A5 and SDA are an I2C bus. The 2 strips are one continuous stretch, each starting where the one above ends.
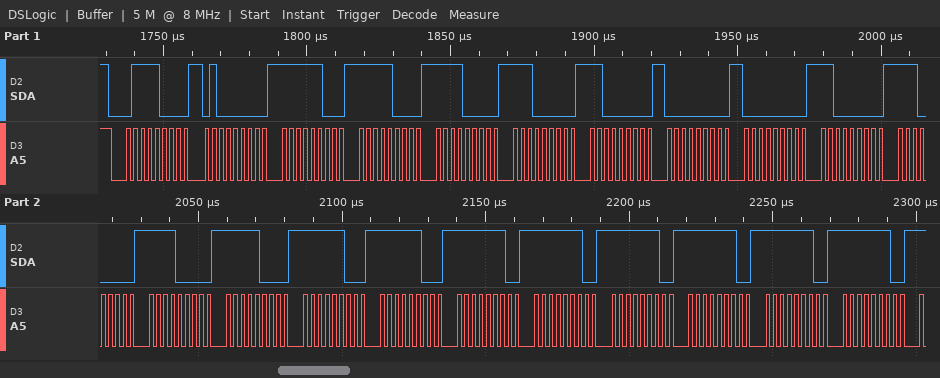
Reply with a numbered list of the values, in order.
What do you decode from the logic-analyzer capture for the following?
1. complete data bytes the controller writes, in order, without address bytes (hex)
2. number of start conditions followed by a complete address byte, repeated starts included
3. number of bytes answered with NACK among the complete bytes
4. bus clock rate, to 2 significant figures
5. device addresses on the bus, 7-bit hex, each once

1. 40 FC F8 F0 E0 C0 00 00 C0 E0 F0 F8 FC FC FE FE FE FE FE FE
2. 1
3. 0
4. 400 kHz
5. 0x3C
